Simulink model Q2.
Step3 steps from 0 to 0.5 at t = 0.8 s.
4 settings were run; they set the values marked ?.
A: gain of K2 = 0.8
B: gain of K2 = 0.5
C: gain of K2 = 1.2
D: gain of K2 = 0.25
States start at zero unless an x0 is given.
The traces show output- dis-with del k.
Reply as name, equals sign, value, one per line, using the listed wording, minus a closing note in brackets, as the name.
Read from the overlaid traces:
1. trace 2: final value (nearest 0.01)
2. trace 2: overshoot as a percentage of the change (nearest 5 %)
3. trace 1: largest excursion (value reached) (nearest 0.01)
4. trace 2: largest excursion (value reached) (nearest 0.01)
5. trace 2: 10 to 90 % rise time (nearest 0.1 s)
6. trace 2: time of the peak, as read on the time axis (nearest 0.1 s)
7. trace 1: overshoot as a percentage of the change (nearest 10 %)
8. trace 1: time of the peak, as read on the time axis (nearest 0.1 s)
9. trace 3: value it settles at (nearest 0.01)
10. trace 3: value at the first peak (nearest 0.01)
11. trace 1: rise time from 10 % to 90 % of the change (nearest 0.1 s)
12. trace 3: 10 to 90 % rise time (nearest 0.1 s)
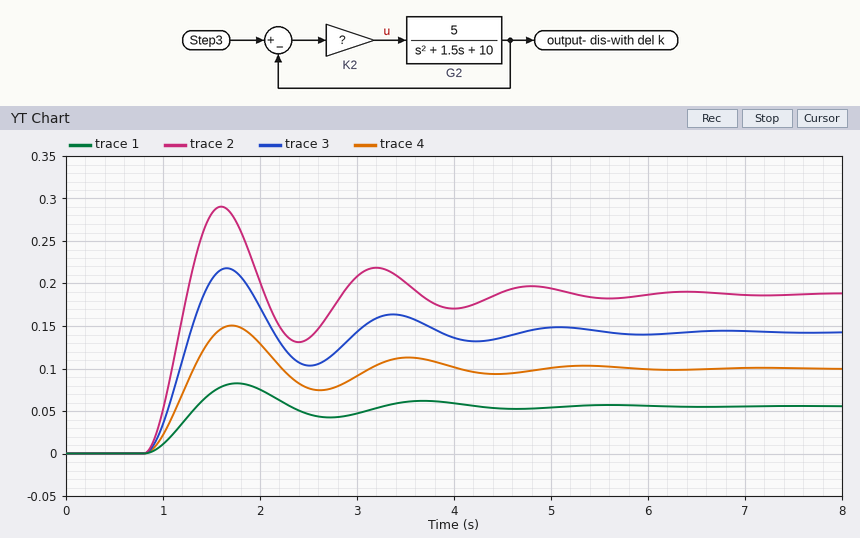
trace 2: final value = 0.19
trace 2: overshoot as a percentage of the change = 55 %
trace 1: largest excursion (value reached) = 0.08
trace 2: largest excursion (value reached) = 0.29
trace 2: 10 to 90 % rise time = 0.3 s
trace 2: time of the peak, as read on the time axis = 1.6 s
trace 1: overshoot as a percentage of the change = 50 %
trace 1: time of the peak, as read on the time axis = 1.8 s
trace 3: value it settles at = 0.14
trace 3: value at the first peak = 0.22
trace 1: rise time from 10 % to 90 % of the change = 0.4 s
trace 3: 10 to 90 % rise time = 0.3 s
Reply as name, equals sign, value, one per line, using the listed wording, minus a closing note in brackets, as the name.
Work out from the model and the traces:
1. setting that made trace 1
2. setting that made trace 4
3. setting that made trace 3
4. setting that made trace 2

setting that made trace 1 = D
setting that made trace 4 = B
setting that made trace 3 = A
setting that made trace 2 = C
